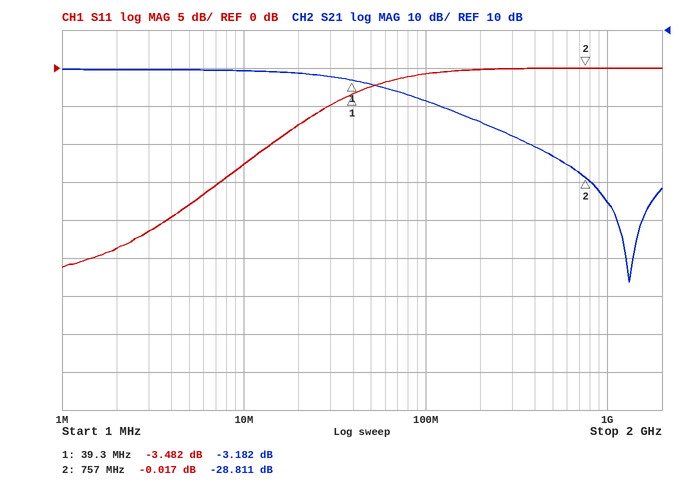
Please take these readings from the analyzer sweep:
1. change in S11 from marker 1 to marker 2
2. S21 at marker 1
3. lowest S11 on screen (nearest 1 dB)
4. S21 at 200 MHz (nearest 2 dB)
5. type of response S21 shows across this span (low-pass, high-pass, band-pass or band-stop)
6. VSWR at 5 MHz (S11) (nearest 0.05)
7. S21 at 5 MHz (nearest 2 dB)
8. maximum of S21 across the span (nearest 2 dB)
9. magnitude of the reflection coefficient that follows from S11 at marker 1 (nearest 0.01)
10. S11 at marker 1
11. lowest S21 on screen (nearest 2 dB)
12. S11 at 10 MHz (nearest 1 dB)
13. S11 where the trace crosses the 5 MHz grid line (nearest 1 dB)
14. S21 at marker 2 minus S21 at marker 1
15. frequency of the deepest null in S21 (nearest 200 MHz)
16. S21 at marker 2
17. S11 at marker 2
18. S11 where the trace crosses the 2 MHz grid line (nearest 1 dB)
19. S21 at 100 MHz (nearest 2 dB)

3.465 dB
-3.182 dB
-26 dB
-14 dB
low-pass
1.30
0 dB
0 dB
0.67
-3.482 dB
-56 dB
-13 dB
-18 dB
-25.629 dB
1.4 GHz
-28.811 dB
-0.017 dB
-24 dB
-8 dB
